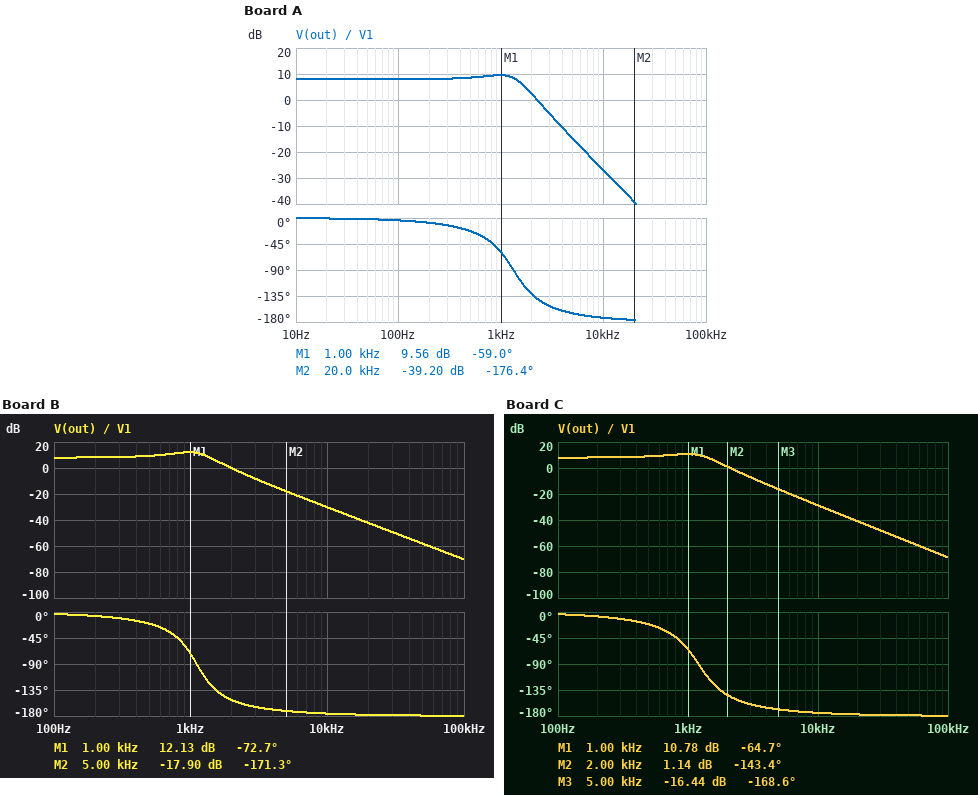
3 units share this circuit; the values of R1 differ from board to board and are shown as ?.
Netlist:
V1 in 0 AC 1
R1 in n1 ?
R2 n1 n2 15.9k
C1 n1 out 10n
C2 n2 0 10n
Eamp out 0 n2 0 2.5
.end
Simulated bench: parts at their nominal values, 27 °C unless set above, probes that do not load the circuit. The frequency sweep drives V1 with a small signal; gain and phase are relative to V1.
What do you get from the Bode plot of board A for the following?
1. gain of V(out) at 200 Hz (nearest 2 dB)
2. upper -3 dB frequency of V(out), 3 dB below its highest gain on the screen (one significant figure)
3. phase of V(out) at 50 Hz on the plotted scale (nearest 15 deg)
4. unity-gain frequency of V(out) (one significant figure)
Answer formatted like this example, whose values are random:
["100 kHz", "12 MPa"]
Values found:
["8 dB", "2 kHz", "0 deg", "2 kHz"]
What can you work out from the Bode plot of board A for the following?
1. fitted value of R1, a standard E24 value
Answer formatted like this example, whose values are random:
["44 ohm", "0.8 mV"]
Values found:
["9.1 kΩ"]
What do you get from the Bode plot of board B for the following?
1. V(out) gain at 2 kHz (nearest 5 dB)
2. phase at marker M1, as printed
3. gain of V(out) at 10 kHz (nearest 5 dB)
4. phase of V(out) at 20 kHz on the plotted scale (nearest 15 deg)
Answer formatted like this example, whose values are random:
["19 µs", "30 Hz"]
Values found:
["0 dB", "-72.7 deg", "-30 dB", "-180 deg"]
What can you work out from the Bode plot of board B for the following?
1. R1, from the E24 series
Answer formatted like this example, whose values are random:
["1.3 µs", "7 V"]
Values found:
["13 kΩ"]
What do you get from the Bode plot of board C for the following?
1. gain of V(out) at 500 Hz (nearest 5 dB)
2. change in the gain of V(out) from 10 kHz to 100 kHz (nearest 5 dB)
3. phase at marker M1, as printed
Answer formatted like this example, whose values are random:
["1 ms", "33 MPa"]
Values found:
["10 dB", "-40 dB", "-64.7 deg"]
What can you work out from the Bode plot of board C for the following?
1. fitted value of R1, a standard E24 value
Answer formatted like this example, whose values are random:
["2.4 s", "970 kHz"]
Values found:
["11 kΩ"]
